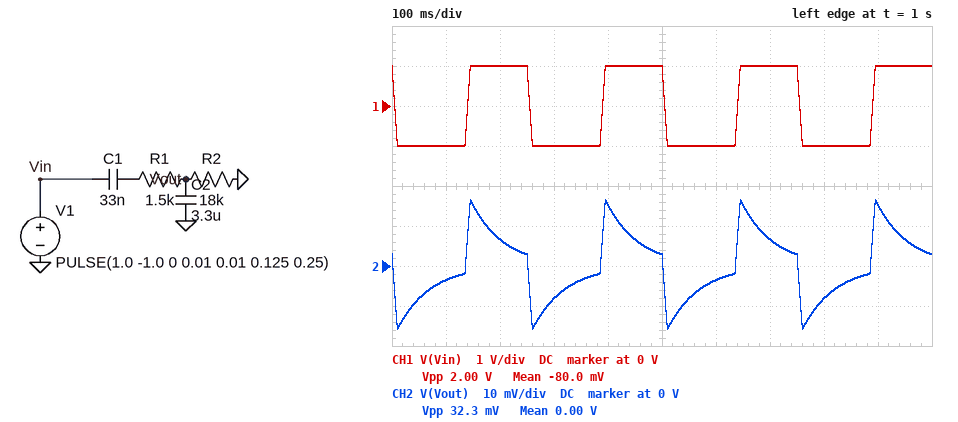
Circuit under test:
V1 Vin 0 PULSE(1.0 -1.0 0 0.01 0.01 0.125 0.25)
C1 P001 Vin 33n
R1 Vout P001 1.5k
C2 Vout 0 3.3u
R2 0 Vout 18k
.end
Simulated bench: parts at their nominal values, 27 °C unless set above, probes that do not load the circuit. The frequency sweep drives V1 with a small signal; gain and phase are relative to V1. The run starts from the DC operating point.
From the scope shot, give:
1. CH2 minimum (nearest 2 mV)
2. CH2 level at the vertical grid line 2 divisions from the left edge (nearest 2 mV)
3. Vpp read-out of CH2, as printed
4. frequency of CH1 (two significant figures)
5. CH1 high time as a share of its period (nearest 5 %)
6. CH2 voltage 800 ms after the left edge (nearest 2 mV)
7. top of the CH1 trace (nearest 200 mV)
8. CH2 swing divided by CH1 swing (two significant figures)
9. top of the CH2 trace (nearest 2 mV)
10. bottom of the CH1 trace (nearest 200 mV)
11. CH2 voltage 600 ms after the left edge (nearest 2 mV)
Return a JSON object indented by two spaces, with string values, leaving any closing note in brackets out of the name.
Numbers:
{
  "CH2 minimum": "-16 mV",
  "CH2 level at the vertical grid line 2 divisions from the left edge": "6 mV",
  "Vpp read-out of CH2, as printed": "32.3 mV",
  "frequency of CH1": "4.0 Hz",
  "CH1 high time as a share of its period": "45 %",
  "CH2 voltage 800 ms after the left edge": "-8 mV",
  "top of the CH1 trace": "1.0 V",
  "CH2 swing divided by CH1 swing": "0.016",
  "top of the CH2 trace": "16 mV",
  "bottom of the CH1 trace": "-1.0 V",
  "CH2 voltage 600 ms after the left edge": "-4 mV"
}
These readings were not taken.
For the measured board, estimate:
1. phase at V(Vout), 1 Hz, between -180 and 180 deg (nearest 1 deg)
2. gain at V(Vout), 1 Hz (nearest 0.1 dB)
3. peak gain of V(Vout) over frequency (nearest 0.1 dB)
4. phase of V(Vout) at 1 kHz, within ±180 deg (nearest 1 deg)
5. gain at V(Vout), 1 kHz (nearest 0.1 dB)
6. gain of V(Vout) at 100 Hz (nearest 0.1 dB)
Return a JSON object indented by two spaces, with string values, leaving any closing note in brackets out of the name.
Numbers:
{
  "phase at V(Vout), 1 Hz, between -180 and 180 deg": "69 deg",
  "gain at V(Vout), 1 Hz": "-49.1 dB",
  "peak gain of V(Vout) over frequency": "-40.1 dB",
  "phase of V(Vout) at 1 kHz, within ±180 deg": "-17 deg",
  "gain at V(Vout), 1 kHz": "-40.5 dB",
  "gain of V(Vout) at 100 Hz": "-40.1 dB"
}
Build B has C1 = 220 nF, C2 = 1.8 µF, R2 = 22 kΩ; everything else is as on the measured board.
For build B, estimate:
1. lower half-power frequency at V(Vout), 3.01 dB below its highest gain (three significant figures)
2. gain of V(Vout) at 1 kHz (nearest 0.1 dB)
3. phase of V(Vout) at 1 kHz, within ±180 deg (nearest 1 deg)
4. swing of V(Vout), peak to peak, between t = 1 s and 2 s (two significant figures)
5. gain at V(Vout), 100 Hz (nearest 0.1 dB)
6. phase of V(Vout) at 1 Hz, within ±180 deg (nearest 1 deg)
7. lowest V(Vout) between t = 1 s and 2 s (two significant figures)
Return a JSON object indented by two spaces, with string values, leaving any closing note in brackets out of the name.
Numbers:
{
  "lower half-power frequency at V(Vout), 3.01 dB below its highest gain": "3.53 Hz",
  "gain of V(Vout) at 1 kHz": "-25.7 dB",
  "phase of V(Vout) at 1 kHz, within ±180 deg": "-61 deg",
  "swing of V(Vout), peak to peak, between t = 1 s and 2 s": "360 mV",
  "gain at V(Vout), 100 Hz": "-19.4 dB",
  "phase of V(Vout) at 1 Hz, within ±180 deg": "74 deg",
  "lowest V(Vout) between t = 1 s and 2 s": "-180 mV"
}
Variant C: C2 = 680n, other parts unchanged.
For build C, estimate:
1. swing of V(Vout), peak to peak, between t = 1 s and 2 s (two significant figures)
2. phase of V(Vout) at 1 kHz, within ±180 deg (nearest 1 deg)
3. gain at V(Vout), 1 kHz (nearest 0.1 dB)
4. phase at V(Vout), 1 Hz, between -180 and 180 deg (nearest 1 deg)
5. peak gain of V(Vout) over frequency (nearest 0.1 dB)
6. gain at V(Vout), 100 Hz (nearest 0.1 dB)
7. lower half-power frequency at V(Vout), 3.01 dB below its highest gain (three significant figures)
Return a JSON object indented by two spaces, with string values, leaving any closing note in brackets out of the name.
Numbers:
{
  "swing of V(Vout), peak to peak, between t = 1 s and 2 s": "130 mV",
  "phase of V(Vout) at 1 kHz, within ±180 deg": "-16 deg",
  "gain at V(Vout), 1 kHz": "-27.1 dB",
  "phase at V(Vout), 1 Hz, between -180 and 180 deg": "85 deg",
  "peak gain of V(Vout) over frequency": "-26.7 dB",
  "gain at V(Vout), 100 Hz": "-26.8 dB",
  "lower half-power frequency at V(Vout), 3.01 dB below its highest gain": "12.3 Hz"
}
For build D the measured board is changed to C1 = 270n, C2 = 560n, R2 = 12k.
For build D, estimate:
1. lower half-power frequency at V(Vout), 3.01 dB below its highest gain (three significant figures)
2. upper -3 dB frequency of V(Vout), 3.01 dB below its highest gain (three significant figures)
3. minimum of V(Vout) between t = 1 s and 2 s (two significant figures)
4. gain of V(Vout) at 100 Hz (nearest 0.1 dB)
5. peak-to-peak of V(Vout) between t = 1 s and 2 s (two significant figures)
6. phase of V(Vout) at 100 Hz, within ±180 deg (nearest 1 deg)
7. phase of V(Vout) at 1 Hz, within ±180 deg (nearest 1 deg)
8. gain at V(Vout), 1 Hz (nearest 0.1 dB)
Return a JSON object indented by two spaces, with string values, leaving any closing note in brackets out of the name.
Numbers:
{
  "lower half-power frequency at V(Vout), 3.01 dB below its highest gain": "15.0 Hz",
  "upper -3 dB frequency of V(Vout), 3.01 dB below its highest gain": "621 Hz",
  "minimum of V(Vout) between t = 1 s and 2 s": "-400 mV",
  "gain of V(Vout) at 100 Hz": "-10.1 dB",
  "peak-to-peak of V(Vout) between t = 1 s and 2 s": "800 mV",
  "phase of V(Vout) at 100 Hz, within ±180 deg": "-1 deg",
  "phase of V(Vout) at 1 Hz, within ±180 deg": "86 deg",
  "gain at V(Vout), 1 Hz": "-33.8 dB"
}
